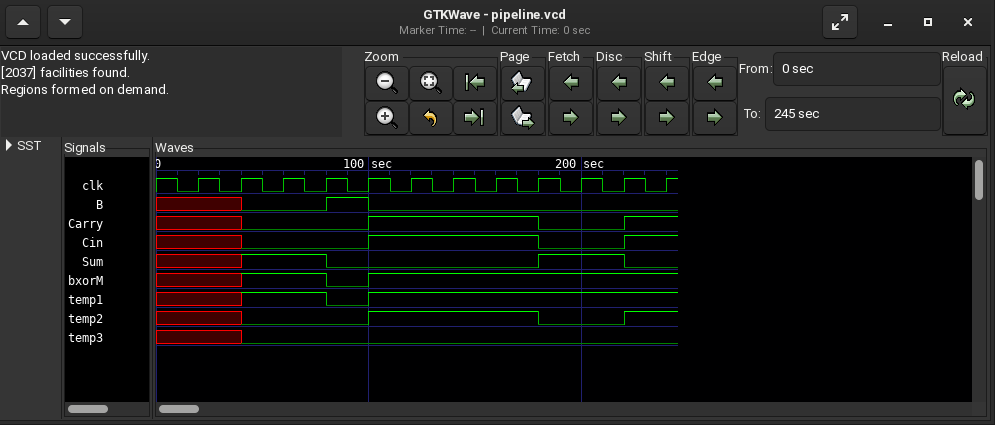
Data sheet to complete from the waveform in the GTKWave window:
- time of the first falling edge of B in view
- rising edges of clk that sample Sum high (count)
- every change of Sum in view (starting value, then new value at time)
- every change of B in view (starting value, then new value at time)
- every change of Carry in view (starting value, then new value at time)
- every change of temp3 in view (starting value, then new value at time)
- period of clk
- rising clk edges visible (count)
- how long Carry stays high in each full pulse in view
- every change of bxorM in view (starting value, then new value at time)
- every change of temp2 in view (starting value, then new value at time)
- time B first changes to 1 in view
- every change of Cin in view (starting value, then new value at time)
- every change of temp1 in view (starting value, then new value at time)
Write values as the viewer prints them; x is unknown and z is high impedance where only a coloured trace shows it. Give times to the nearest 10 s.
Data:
100 s
4
x, 1 at 40 s, 0 at 80 s, 1 at 180 s, 0 at 220 s
x, 0 at 40 s, 1 at 80 s, 0 at 100 s
x, 0 at 40 s, 1 at 100 s, 0 at 180 s, 1 at 220 s
x, 0 at 40 s
20 s
12
80 s
x, 1 at 40 s, 0 at 80 s, 1 at 100 s
x, 0 at 40 s, 1 at 100 s, 0 at 180 s, 1 at 220 s
80 s
x, 0 at 40 s, 1 at 100 s, 0 at 180 s, 1 at 220 s
x, 1 at 40 s, 0 at 80 s, 1 at 100 s
